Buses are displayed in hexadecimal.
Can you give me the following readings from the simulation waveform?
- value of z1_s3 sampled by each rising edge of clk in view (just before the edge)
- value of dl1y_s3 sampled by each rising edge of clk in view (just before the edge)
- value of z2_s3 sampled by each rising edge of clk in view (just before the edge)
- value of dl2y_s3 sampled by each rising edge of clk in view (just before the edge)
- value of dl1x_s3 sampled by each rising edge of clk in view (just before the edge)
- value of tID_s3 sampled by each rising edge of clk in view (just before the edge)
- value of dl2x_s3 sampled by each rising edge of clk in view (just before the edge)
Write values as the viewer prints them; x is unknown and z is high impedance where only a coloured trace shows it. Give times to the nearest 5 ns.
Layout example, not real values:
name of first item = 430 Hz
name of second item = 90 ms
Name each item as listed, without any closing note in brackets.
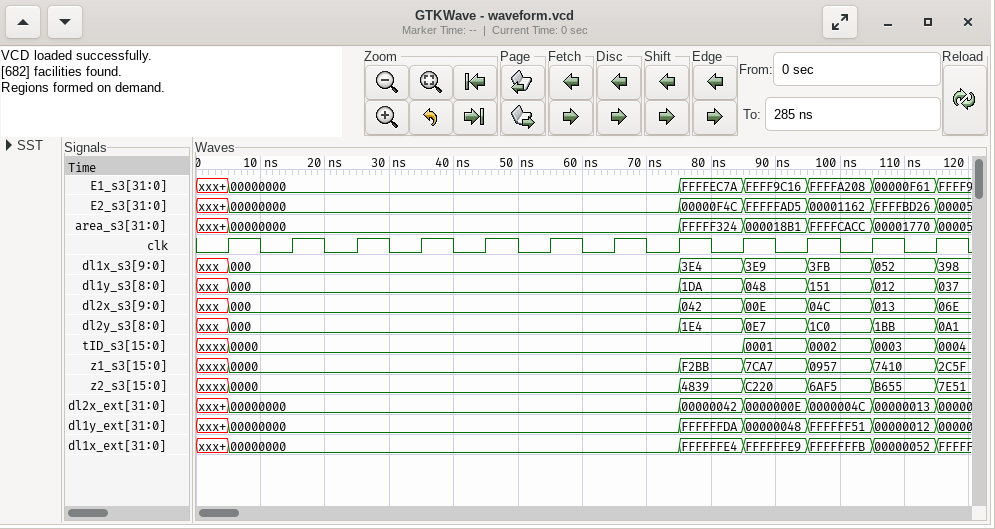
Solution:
value of z1_s3 sampled by each rising edge of clk in view = xxxx, 0000, 0000, 0000, 0000, 0000, 0000, 0000, F2BB, 7CA7, 0957, 7410
value of dl1y_s3 sampled by each rising edge of clk in view = xxx, 000, 000, 000, 000, 000, 000, 000, 1DA, 048, 151, 012
value of z2_s3 sampled by each rising edge of clk in view = xxxx, 0000, 0000, 0000, 0000, 0000, 0000, 0000, 4839, C220, 6AF5, B655
value of dl2y_s3 sampled by each rising edge of clk in view = xxx, 000, 000, 000, 000, 000, 000, 000, 1E4, 0E7, 1C0, 1BB
value of dl1x_s3 sampled by each rising edge of clk in view = xxx, 000, 000, 000, 000, 000, 000, 000, 3E4, 3E9, 3FB, 052
value of tID_s3 sampled by each rising edge of clk in view = xxxx, 0000, 0000, 0000, 0000, 0000, 0000, 0000, 0000, 0001, 0002, 0003
value of dl2x_s3 sampled by each rising edge of clk in view = xxx, 000, 000, 000, 000, 000, 000, 000, 042, 00E, 04C, 013
